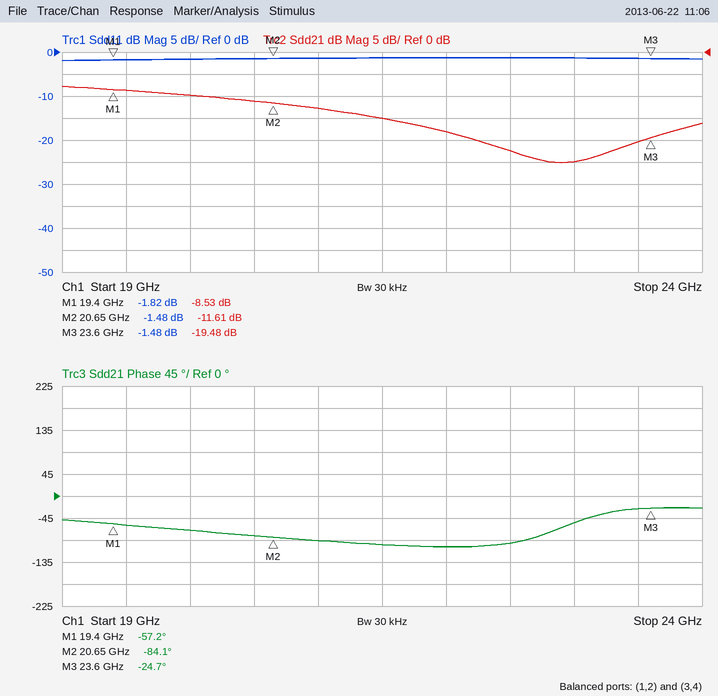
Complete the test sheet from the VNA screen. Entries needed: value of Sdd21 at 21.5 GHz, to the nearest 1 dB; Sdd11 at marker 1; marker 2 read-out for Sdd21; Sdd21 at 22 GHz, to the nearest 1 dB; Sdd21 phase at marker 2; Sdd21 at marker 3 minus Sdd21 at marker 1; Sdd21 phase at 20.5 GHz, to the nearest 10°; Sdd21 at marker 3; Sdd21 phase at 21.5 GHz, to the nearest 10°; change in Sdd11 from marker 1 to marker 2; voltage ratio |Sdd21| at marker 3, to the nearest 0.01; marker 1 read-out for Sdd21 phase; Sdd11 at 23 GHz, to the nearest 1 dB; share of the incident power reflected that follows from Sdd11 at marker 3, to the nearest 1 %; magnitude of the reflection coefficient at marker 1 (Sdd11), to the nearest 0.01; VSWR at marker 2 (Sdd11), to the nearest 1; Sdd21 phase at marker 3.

-15 dB
-1.82 dB
-11.61 dB
-18 dB
-84.1°
-10.95 dB
-80°
-19.48 dB
-100°
0.34 dB
0.11
-57.2°
-1 dB
71 %
0.81
12
-24.7°
